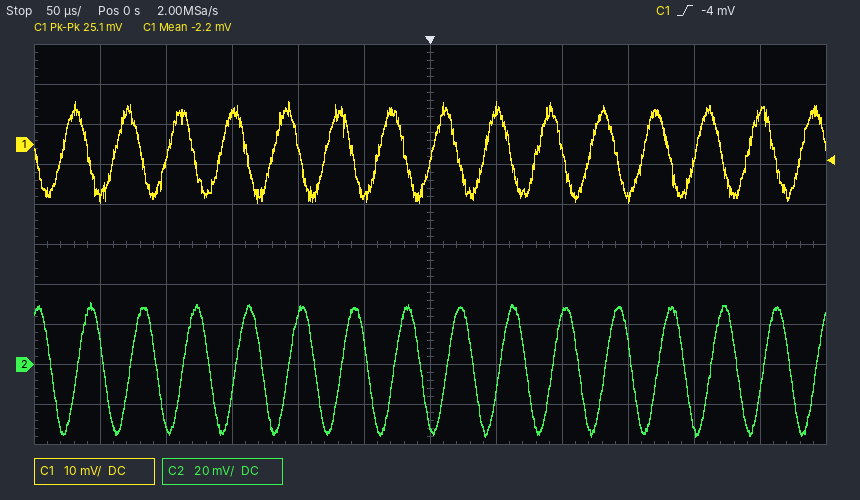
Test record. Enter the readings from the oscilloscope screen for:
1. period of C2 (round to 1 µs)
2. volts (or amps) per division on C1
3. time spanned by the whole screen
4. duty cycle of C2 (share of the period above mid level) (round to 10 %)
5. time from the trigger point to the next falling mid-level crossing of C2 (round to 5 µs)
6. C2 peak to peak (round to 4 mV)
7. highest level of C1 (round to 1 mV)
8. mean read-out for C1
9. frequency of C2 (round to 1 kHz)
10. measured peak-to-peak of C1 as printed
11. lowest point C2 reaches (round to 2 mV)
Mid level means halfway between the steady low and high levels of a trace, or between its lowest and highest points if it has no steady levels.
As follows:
40 µs
10 mV
600 µs
50 %
35 µs
68 mV
11 mV
-2.2 mV
25 kHz
25.1 mV
-36 mV
